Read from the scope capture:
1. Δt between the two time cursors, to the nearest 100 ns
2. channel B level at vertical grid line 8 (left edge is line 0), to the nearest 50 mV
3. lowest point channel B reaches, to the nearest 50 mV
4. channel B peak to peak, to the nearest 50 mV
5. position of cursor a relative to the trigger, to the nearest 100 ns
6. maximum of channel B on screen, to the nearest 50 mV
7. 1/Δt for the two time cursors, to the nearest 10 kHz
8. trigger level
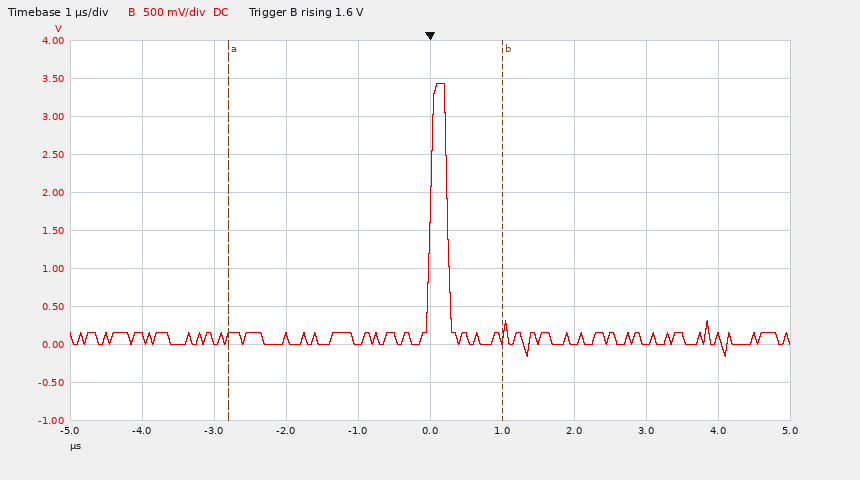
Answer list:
3.8 µs
0 mV
-150 mV
3.60 V
-2.8 µs
3.45 V
260 kHz
1.6 V
